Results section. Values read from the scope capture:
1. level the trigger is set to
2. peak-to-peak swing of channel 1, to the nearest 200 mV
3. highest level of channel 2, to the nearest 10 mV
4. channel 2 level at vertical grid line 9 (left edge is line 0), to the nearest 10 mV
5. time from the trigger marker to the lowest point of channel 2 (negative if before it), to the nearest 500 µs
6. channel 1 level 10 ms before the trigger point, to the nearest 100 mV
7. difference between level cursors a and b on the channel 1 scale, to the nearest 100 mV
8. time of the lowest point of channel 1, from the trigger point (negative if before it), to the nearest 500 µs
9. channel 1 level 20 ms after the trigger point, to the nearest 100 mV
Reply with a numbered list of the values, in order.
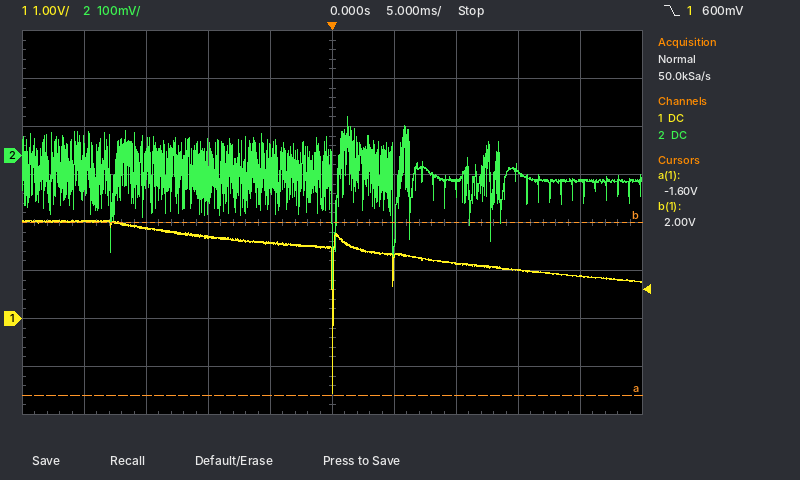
1. 600 mV
2. 3.6 V
3. 80 mV
4. -50 mV
5. 0.0 ms
6. 1.7 V
7. 3.6 V
8. 0.0 ms
9. 900 mV
